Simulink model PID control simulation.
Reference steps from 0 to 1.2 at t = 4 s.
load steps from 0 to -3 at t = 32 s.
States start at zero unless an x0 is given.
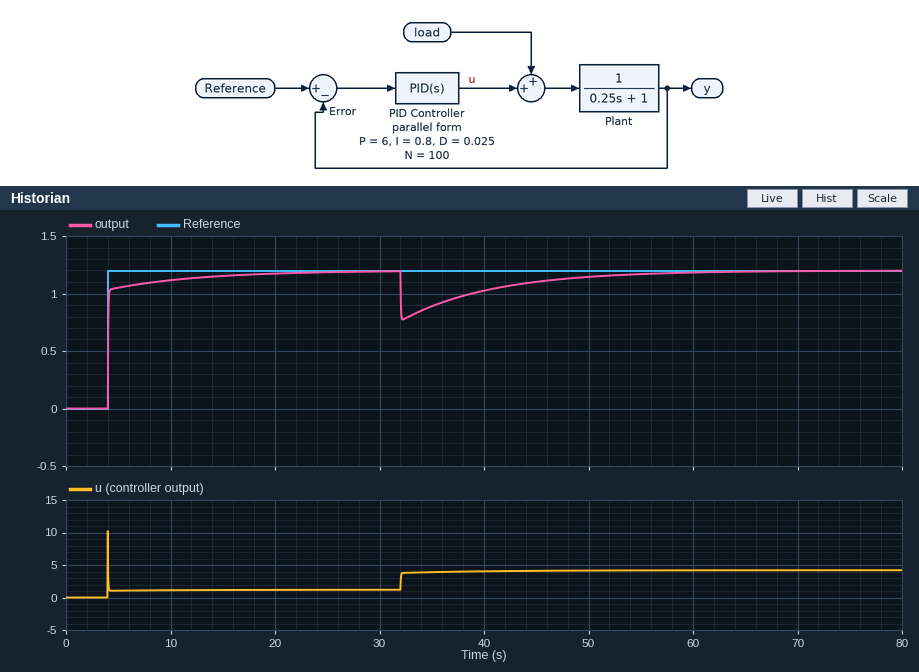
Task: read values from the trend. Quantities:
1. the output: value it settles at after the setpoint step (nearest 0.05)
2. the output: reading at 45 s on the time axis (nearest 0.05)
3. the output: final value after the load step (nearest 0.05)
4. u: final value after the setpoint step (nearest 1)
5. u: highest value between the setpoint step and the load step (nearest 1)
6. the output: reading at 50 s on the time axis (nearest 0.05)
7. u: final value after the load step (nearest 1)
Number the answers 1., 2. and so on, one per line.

1. 1.20
2. 1.10
3. 1.20
4. 1
5. 10
6. 1.15
7. 4
